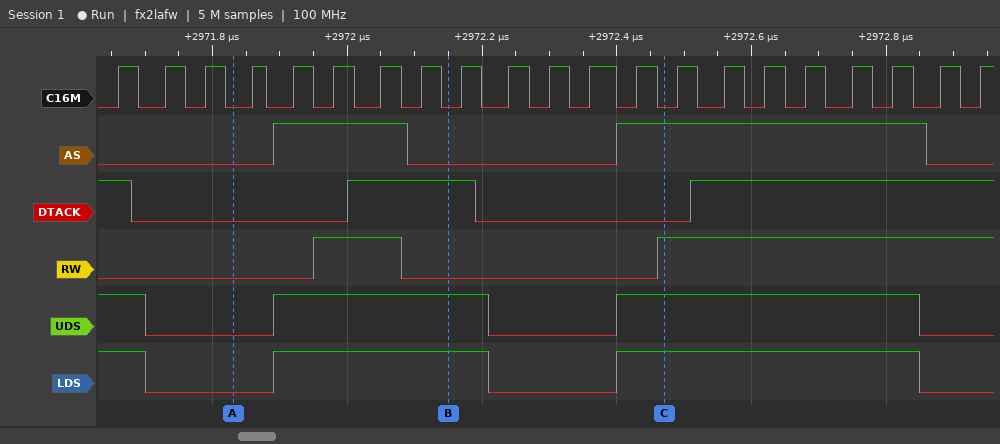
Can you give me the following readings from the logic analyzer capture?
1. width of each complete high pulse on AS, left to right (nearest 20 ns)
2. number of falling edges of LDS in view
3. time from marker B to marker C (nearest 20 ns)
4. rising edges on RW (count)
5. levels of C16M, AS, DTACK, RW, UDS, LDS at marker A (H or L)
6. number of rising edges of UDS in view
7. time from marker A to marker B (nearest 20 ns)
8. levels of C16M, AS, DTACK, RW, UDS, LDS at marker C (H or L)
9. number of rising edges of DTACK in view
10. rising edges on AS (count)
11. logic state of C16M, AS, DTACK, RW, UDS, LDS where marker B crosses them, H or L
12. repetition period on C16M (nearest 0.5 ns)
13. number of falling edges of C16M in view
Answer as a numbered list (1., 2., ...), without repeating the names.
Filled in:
1. 200 ns, 460 ns
2. 3
3. 320 ns
4. 2
5. C16M=L, AS=L, DTACK=L, RW=L, UDS=L, LDS=L
6. 2
7. 320 ns
8. C16M=L, AS=H, DTACK=L, RW=H, UDS=H, LDS=H
9. 2
10. 2
11. C16M=L, AS=L, DTACK=H, RW=L, UDS=H, LDS=H
12. 64 ns
13. 20
